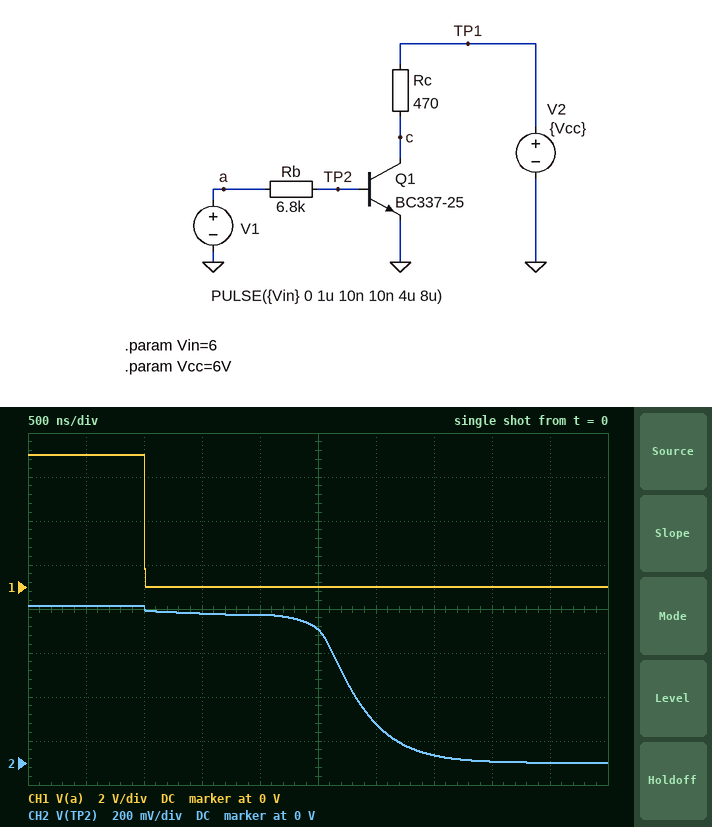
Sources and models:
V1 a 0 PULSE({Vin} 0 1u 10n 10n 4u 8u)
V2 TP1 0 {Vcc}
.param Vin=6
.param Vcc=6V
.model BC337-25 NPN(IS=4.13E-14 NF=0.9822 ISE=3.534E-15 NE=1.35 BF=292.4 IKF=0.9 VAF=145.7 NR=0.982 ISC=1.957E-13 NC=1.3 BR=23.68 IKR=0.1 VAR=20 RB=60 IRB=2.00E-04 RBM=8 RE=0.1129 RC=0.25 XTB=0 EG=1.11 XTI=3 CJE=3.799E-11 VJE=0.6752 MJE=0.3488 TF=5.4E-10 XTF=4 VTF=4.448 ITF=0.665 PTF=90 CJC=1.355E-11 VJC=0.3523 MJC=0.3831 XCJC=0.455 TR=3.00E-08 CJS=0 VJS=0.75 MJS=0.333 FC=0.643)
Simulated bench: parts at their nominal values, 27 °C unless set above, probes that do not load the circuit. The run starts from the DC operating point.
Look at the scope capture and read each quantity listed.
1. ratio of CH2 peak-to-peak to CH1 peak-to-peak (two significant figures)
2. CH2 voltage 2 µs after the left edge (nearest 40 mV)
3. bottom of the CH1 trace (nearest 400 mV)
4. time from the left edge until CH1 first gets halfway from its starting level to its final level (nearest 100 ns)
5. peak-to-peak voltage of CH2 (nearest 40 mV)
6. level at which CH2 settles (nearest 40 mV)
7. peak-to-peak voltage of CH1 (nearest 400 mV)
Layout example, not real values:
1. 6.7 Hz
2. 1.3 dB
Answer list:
1. 0.12
2. 680 mV
3. 0 V
4. 1.0 µs
5. 720 mV
6. 0 V
7. 6.0 V
